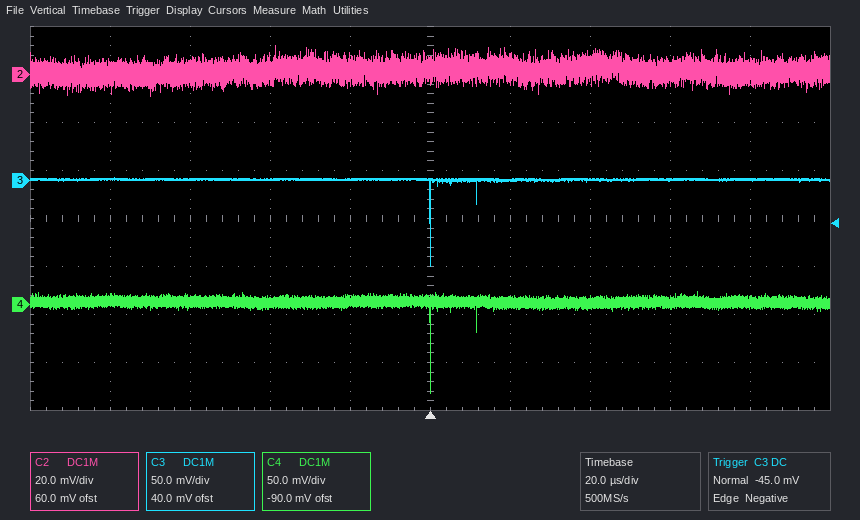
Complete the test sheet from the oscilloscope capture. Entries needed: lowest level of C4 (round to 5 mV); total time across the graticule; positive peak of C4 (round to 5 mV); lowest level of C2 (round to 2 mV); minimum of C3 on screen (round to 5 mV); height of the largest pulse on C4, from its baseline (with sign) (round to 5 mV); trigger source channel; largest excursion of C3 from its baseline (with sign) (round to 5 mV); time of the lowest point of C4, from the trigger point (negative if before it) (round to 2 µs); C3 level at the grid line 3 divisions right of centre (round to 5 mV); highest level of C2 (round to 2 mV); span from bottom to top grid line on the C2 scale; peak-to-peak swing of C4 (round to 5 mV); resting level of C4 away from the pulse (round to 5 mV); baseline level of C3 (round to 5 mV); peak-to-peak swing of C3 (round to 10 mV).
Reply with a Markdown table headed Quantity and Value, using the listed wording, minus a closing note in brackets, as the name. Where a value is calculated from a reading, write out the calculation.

| Quantity | Value |
|---|---|
| lowest level of C4 | -90 mV |
| total time across the graticule | 200 µs |
| positive peak of C4 | 15 mV |
| lowest level of C2 | -10 mV |
| minimum of C3 on screen | -90 mV |
| height of the largest pulse on C4, from its baseline (with sign) | -90 mV − (5 mV) = -95 mV |
| trigger source channel | C3 |
| largest excursion of C3 from its baseline (with sign) | -90 mV − (0 mV) = -90 mV |
| time of the lowest point of C4, from the trigger point (negative if before it) | 0 µs |
| C3 level at the grid line 3 divisions right of centre | 0 mV |
| highest level of C2 | 12 mV |
| span from bottom to top grid line on the C2 scale | 160 mV |
| peak-to-peak swing of C4 | 15 mV − (-90 mV) = 105 mV |
| resting level of C4 away from the pulse | 5 mV |
| baseline level of C3 | 0 mV |
| peak-to-peak swing of C3 | 90 mV |
